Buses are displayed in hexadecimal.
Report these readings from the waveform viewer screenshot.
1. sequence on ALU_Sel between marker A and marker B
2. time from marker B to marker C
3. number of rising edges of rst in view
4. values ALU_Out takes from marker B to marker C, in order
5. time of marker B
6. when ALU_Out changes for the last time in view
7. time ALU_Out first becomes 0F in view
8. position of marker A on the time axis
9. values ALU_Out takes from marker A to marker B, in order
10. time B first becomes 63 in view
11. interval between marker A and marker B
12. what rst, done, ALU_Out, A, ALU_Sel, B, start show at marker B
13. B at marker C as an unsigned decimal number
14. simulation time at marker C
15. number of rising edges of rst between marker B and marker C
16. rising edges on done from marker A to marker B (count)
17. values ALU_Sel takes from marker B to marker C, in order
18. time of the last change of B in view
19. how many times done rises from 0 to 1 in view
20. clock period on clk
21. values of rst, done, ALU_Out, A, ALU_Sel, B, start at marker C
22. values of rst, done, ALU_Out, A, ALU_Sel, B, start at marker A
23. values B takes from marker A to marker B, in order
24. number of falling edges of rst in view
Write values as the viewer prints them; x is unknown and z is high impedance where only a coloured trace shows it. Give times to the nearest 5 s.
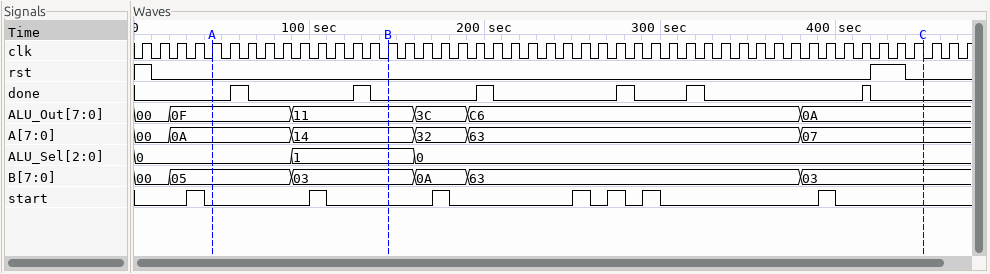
0, 1
305 s
1
11, 3C, C6, 0A
145 s
380 s
20 s
45 s
0F, 11
190 s
100 s
rst=0, done=0, ALU_Out=11, A=14, ALU_Sel=1, B=03, start=0
3
450 s
1
2
1, 0
380 s
6
10 s
rst=0, done=0, ALU_Out=0A, A=07, ALU_Sel=0, B=03, start=0
rst=0, done=0, ALU_Out=0F, A=0A, ALU_Sel=0, B=05, start=0
05, 03
2
